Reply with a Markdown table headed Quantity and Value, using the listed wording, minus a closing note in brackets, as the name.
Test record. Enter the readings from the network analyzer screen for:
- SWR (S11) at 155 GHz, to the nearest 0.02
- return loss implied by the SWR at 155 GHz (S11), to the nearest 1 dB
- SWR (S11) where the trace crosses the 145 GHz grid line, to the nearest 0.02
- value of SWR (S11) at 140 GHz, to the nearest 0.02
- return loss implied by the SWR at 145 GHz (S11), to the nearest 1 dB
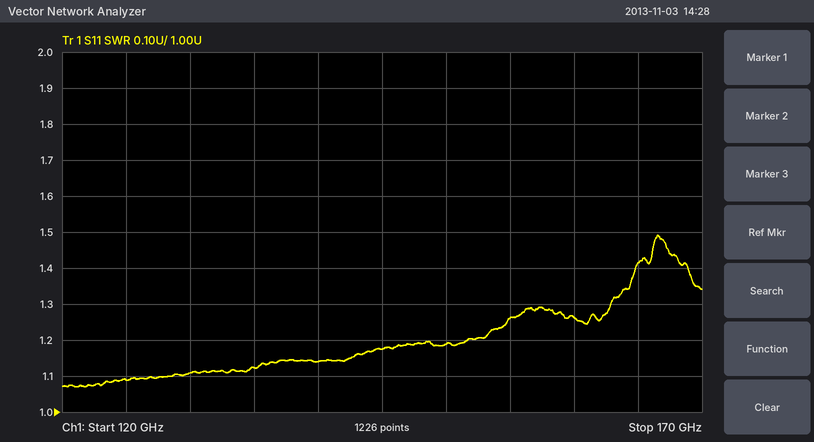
| Quantity | Value |
|---|---|
| SWR (S11) at 155 GHz, to the nearest 0.02 | 1.26 |
| return loss implied by the SWR at 155 GHz (S11), to the nearest 1 dB | 19 dB |
| SWR (S11) where the trace crosses the 145 GHz grid line, to the nearest 0.02 | 1.18 |
| value of SWR (S11) at 140 GHz, to the nearest 0.02 | 1.14 |
| return loss implied by the SWR at 145 GHz (S11), to the nearest 1 dB | 22 dB |
